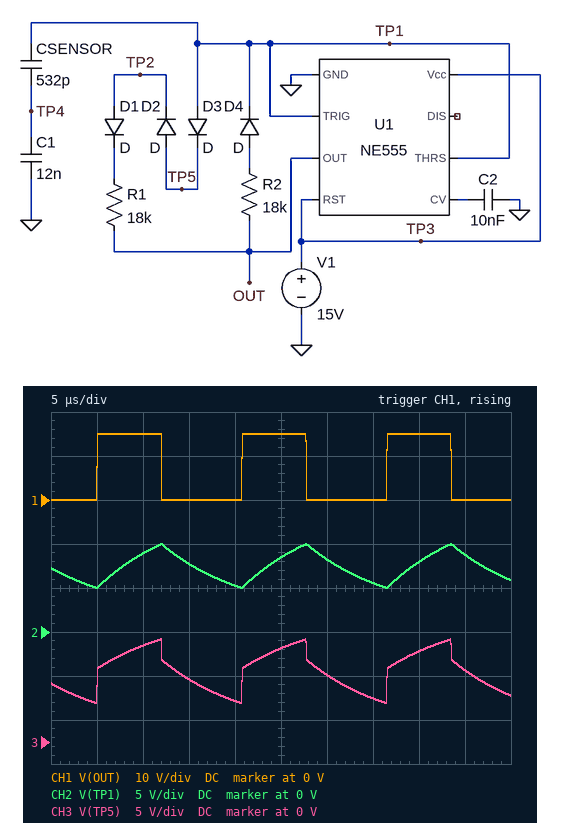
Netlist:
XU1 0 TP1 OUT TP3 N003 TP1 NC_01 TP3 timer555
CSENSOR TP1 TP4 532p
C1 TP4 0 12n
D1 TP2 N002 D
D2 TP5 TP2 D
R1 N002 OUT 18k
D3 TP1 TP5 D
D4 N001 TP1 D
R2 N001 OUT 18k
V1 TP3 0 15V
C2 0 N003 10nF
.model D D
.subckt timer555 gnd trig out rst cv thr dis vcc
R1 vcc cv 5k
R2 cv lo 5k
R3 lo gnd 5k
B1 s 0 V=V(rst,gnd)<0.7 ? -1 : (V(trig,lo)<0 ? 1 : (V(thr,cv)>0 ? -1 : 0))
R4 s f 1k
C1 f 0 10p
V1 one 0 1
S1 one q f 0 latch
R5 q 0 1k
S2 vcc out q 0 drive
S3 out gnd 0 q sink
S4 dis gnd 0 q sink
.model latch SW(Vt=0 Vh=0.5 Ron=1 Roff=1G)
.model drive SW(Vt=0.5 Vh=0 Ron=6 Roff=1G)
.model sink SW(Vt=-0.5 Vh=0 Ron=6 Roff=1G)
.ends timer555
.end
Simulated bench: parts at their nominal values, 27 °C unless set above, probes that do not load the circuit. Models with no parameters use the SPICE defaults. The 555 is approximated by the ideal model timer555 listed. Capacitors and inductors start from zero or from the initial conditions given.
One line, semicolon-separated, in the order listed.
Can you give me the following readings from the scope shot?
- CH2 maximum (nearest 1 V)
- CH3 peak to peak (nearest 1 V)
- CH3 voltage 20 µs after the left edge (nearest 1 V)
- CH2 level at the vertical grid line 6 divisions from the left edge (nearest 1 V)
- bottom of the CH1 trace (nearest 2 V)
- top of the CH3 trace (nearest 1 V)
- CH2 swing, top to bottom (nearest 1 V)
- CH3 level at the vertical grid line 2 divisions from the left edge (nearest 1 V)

10 V; 7 V; 5 V; 8 V; 0 V; 12 V; 5 V; 11 V
